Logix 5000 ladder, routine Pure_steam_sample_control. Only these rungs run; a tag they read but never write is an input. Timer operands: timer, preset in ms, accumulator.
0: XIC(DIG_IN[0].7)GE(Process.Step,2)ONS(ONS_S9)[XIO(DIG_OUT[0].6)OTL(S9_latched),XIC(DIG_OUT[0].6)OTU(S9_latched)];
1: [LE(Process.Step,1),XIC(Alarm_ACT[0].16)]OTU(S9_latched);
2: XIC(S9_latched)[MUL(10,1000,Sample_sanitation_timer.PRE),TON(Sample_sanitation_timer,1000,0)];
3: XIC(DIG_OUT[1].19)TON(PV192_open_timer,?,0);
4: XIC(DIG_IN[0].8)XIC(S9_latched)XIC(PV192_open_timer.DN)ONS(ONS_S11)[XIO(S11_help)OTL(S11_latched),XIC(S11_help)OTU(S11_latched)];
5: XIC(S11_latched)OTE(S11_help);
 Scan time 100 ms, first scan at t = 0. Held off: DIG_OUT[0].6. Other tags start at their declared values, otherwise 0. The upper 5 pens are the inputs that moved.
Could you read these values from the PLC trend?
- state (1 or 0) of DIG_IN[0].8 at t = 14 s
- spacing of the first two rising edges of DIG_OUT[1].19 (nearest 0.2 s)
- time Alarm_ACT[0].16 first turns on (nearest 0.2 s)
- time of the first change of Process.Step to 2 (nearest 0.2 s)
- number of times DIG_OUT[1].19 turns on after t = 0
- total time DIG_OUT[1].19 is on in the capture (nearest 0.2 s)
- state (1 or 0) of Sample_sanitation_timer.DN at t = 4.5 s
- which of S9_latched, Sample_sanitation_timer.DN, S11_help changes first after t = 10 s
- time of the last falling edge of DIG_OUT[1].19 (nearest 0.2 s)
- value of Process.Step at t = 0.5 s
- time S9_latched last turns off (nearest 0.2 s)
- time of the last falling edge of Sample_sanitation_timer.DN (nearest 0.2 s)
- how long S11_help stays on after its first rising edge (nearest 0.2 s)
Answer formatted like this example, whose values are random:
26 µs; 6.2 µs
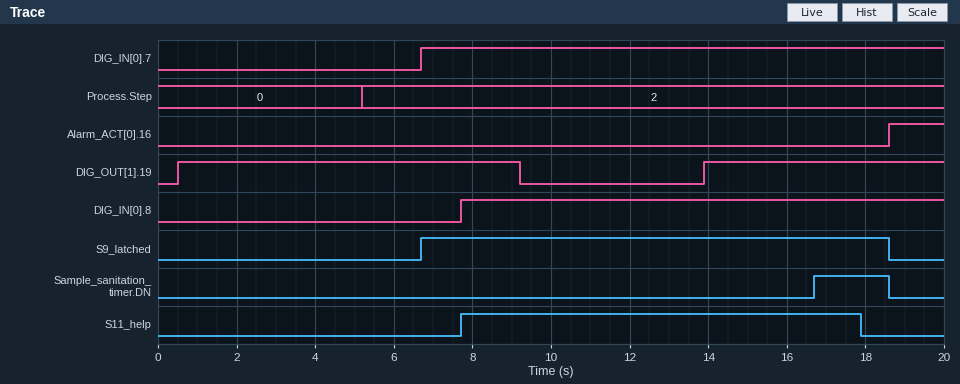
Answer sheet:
1; 13.4 s; 18.6 s; 5.2 s; 2; 14.8 s; 0; Sample_sanitation_timer.DN; 9.2 s; 0; 18.6 s; 18.6 s; 10.2 s
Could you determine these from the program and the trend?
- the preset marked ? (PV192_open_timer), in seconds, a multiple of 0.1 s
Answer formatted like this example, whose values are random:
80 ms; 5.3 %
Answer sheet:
4.0 s
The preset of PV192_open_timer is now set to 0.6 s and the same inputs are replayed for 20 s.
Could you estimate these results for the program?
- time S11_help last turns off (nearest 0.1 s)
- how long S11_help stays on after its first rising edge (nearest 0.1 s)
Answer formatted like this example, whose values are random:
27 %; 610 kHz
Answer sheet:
14.5 s; 6.8 s
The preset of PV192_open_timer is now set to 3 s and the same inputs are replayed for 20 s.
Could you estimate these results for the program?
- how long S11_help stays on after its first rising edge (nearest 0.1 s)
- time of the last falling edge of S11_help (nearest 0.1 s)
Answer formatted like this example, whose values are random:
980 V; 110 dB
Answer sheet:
9.2 s; 16.9 s
